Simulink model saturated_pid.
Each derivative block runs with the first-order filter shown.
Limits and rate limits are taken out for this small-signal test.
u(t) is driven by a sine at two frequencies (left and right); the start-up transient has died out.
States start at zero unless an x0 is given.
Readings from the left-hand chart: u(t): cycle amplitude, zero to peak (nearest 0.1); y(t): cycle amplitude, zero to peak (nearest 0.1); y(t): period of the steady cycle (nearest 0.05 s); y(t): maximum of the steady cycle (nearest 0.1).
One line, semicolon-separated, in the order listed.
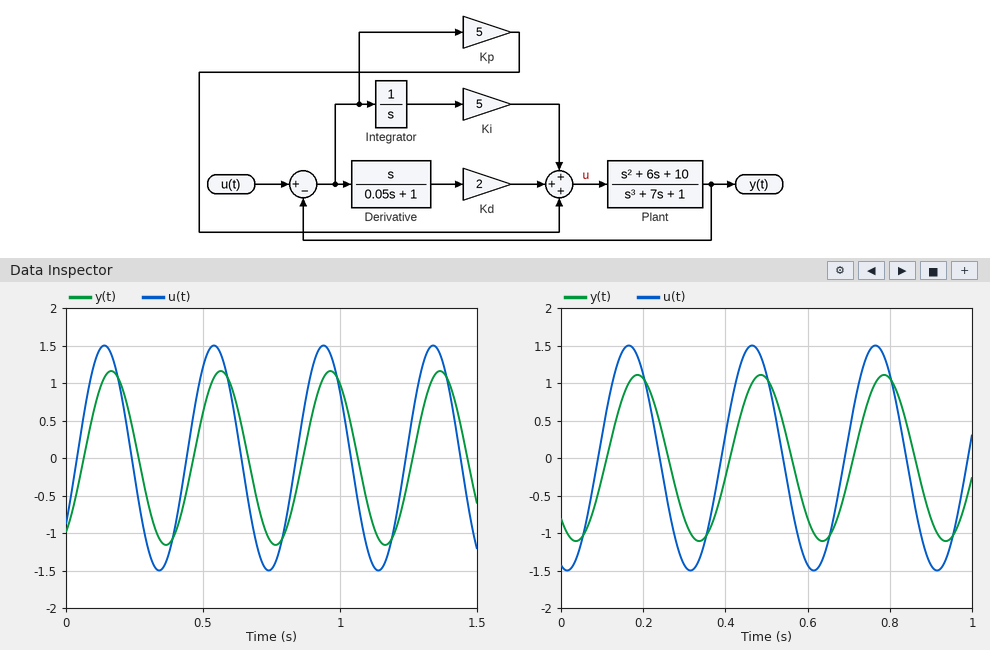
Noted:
1.5; 1.2; 0.40 s; 1.2
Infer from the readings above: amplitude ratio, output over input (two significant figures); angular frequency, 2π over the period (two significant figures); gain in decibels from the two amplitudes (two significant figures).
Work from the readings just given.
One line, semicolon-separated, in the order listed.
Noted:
0.80; 16 rad/s; -1.9 dB
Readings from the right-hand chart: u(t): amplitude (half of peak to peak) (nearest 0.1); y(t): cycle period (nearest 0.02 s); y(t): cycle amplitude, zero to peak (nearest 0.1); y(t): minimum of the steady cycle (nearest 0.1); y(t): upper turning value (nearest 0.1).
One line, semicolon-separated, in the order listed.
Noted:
1.5; 0.30 s; 1.1; -1.1; 1.1
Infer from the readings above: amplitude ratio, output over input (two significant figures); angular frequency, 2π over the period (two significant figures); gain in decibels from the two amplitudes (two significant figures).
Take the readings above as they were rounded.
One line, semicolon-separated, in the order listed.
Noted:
0.73; 21 rad/s; -2.7 dB
